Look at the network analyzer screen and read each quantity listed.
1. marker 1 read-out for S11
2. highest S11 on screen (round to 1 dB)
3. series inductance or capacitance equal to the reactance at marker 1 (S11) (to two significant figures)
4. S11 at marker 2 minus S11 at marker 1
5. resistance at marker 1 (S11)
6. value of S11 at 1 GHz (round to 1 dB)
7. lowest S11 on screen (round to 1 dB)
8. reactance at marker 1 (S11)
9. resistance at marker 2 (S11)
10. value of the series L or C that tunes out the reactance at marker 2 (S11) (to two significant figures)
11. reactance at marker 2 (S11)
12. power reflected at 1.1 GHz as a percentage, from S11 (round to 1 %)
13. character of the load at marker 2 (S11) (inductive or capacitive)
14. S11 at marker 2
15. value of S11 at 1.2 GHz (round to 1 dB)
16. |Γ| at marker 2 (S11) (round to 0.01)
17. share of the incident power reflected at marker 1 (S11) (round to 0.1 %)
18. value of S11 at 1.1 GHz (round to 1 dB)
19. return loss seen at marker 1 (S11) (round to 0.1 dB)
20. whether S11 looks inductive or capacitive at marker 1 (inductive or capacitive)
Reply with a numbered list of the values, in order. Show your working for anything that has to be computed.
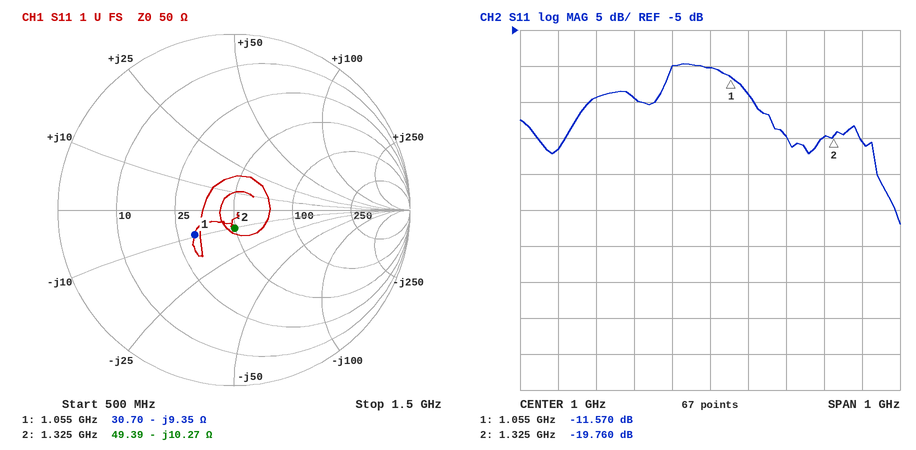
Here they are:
1. -11.570 dB
2. -10 dB
3. C = 1/(2π × 1.055 GHz × 9.35 Ω) ≈ 16 pF
4. -19.76 − (-11.57) = -8.190 dB
5. 30.70 Ω
6. -10 dB
7. -32 dB
8. -9.35 Ω
9. 49.39 Ω
10. L = 10.27 Ω/(2π × 1.325 GHz) ≈ 1.2 nH
11. -10.27 Ω
12. 10^(-14/10) ≈ 4 %
13. capacitive
14. -19.760 dB
15. -20 dB
16. 0.10
17. 10^(-11.57/10) ≈ 7.0 %
18. -14 dB
19. 11.6 dB
20. capacitive
